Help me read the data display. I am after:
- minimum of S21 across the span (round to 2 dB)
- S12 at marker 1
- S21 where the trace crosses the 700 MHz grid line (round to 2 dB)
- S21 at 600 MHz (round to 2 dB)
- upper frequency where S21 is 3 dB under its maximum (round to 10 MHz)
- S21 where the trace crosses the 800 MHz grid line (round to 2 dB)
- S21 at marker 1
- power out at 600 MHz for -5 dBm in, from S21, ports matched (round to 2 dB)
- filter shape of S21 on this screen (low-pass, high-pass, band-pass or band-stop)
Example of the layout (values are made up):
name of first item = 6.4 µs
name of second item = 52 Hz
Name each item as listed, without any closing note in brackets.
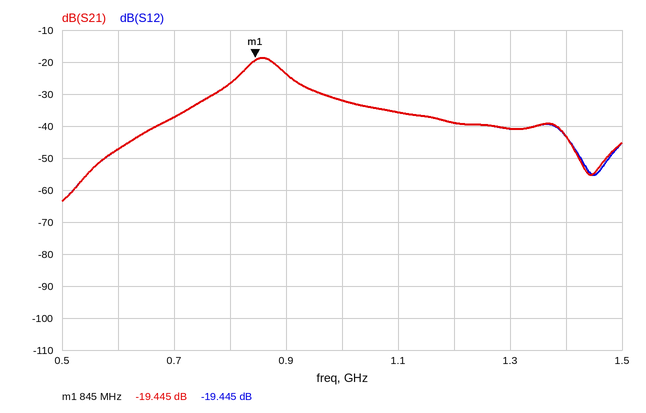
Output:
minimum of S21 across the span = -64 dB
S12 at marker 1 = -19.445 dB
S21 where the trace crosses the 700 MHz grid line = -38 dB
S21 at 600 MHz = -48 dB
upper frequency where S21 is 3 dB under its maximum = 890 MHz
S21 where the trace crosses the 800 MHz grid line = -26 dB
S21 at marker 1 = -19.445 dB
power out at 600 MHz for -5 dBm in, from S21, ports matched = -52 dBm
filter shape of S21 on this screen = band-pass
